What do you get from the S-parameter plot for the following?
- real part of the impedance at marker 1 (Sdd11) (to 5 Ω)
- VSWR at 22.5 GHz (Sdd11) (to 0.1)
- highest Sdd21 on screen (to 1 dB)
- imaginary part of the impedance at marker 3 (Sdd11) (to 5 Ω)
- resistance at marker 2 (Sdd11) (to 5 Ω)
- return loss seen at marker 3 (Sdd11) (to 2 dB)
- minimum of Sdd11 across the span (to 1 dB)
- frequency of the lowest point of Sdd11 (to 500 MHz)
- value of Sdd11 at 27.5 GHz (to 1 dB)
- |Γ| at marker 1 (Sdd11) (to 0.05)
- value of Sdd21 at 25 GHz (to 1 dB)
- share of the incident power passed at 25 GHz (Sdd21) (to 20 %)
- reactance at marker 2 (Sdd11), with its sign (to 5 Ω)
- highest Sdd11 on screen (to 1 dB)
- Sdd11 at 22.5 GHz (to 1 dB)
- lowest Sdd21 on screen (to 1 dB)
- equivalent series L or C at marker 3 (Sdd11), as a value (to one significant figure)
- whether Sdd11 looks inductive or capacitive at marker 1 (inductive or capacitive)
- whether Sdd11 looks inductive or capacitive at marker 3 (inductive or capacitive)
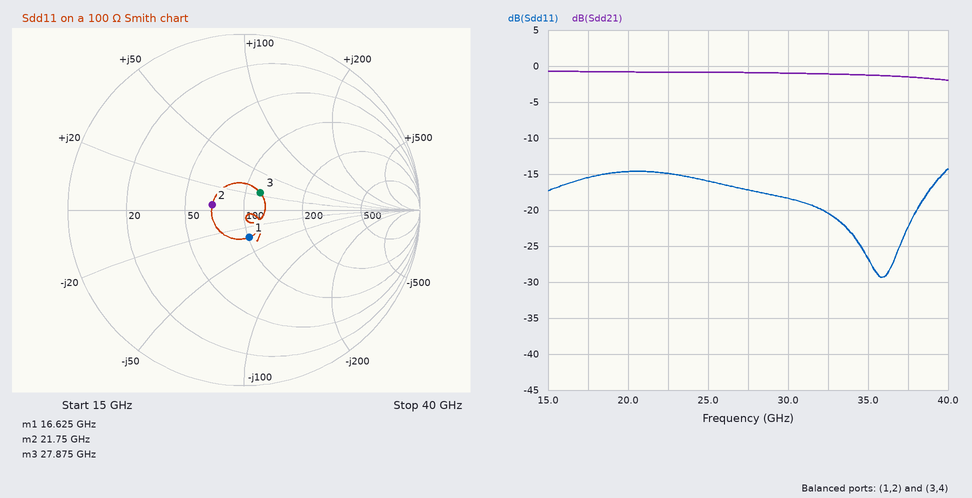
100 Ω
1.4
-1 dB
+25 Ω
70 Ω
18 dB
-29 dB
36.0 GHz
-17 dB
0.15
-1 dB
80 %
+5 Ω
-14 dB
-15 dB
-2 dB
100 pH
capacitive
inductive
